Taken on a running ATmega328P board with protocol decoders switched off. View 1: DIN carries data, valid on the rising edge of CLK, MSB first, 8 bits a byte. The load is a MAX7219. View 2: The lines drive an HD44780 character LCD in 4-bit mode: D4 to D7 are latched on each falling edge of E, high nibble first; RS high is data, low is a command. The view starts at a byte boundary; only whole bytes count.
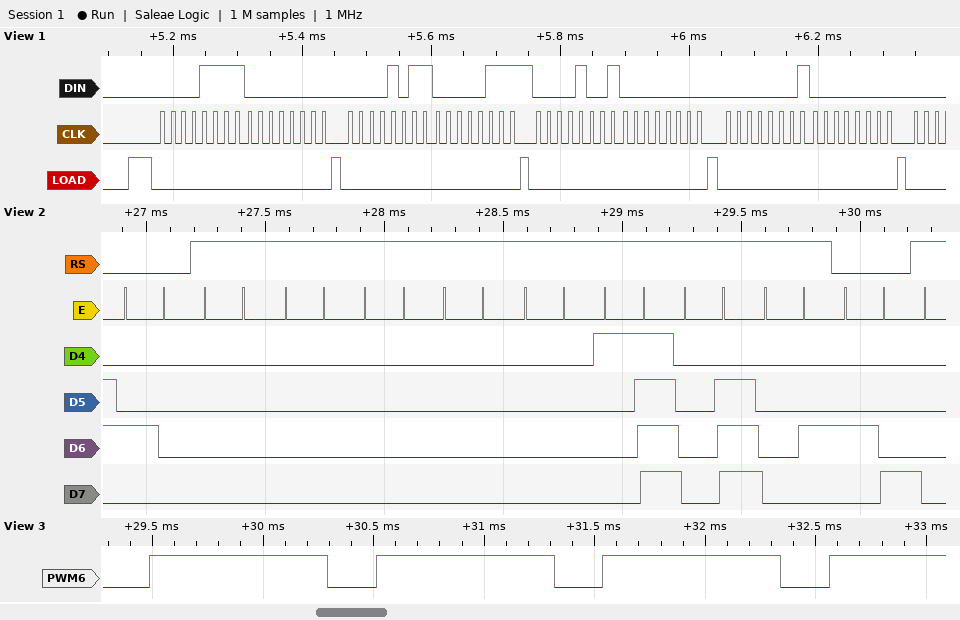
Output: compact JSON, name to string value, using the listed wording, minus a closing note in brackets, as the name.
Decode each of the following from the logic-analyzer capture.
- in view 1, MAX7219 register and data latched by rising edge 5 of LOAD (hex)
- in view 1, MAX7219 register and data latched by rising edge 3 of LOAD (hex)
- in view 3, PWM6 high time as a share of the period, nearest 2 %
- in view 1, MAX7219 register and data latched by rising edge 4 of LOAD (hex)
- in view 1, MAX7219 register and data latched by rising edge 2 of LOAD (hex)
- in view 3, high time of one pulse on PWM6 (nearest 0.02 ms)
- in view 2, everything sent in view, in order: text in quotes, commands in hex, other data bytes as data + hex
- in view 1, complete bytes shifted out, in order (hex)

{"in view 1, MAX7219 register and data latched by rising edge 5 of LOAD": "register 0x1, data 0x00", "in view 1, MAX7219 register and data latched by rising edge 3 of LOAD": "register 0xB, data 0x07", "in view 3, PWM6 high time as a share of the period, nearest 2 %": "78 %", "in view 1, MAX7219 register and data latched by rising edge 4 of LOAD": "register 0x9, data 0x00", "in view 1, MAX7219 register and data latched by rising edge 2 of LOAD": "register 0xF, data 0x00", "in view 3, high time of one pulse on PWM6": "0.80 ms", "in view 2, everything sent in view, in order: text in quotes, commands in hex, other data bytes as data + hex": "0x40 data 00 00 00 00 00 1F 0E 04 0x48", "in view 1, complete bytes shifted out, in order": "0x0F 0x00 0x0B 0x07 0x09 0x00 0x01 0x00"}
